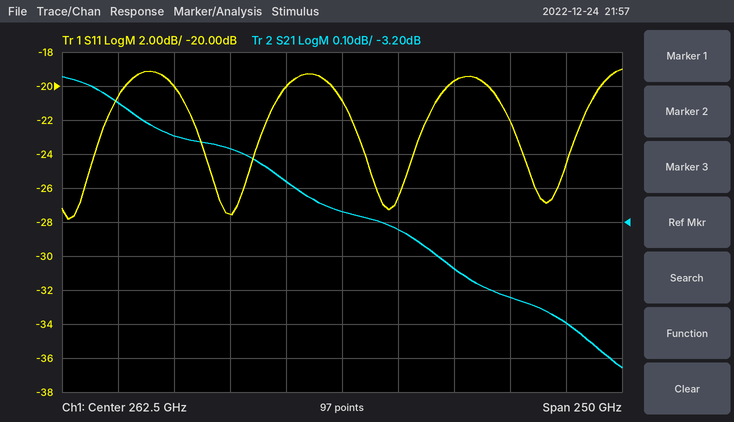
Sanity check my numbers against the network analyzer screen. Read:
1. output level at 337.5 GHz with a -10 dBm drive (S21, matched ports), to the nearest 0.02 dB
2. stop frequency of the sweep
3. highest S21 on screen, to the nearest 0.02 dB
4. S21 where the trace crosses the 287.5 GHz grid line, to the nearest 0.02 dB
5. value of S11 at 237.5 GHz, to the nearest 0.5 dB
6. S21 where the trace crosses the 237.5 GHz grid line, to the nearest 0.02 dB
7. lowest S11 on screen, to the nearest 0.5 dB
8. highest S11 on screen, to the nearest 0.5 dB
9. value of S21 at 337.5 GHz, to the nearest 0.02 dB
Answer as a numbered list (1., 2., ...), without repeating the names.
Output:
1. -13.42 dBm
2. 387.5 GHz
3. -2.78 dB
4. -3.22 dB
5. -20.0 dB
6. -3.08 dB
7. -28.0 dB
8. -19.0 dB
9. -3.42 dB
